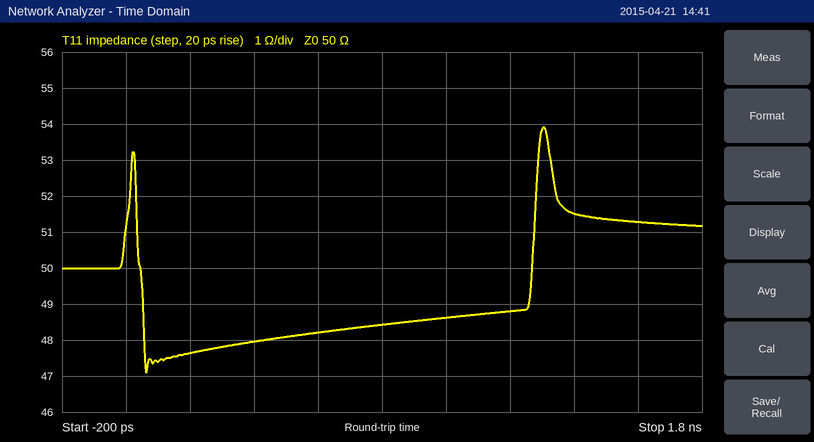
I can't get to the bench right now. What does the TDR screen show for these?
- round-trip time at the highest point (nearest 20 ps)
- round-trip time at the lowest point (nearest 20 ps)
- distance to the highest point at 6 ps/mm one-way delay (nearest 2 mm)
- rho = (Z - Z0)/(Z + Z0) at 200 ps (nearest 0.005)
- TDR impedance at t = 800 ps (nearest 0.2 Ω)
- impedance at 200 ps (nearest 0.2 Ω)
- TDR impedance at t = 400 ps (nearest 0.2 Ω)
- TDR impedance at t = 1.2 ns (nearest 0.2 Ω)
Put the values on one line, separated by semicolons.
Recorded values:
1.30 ns; 60 ps; 108 mm; -0.025; 48.4 Ω; 47.6 Ω; 48.0 Ω; 48.8 Ω
